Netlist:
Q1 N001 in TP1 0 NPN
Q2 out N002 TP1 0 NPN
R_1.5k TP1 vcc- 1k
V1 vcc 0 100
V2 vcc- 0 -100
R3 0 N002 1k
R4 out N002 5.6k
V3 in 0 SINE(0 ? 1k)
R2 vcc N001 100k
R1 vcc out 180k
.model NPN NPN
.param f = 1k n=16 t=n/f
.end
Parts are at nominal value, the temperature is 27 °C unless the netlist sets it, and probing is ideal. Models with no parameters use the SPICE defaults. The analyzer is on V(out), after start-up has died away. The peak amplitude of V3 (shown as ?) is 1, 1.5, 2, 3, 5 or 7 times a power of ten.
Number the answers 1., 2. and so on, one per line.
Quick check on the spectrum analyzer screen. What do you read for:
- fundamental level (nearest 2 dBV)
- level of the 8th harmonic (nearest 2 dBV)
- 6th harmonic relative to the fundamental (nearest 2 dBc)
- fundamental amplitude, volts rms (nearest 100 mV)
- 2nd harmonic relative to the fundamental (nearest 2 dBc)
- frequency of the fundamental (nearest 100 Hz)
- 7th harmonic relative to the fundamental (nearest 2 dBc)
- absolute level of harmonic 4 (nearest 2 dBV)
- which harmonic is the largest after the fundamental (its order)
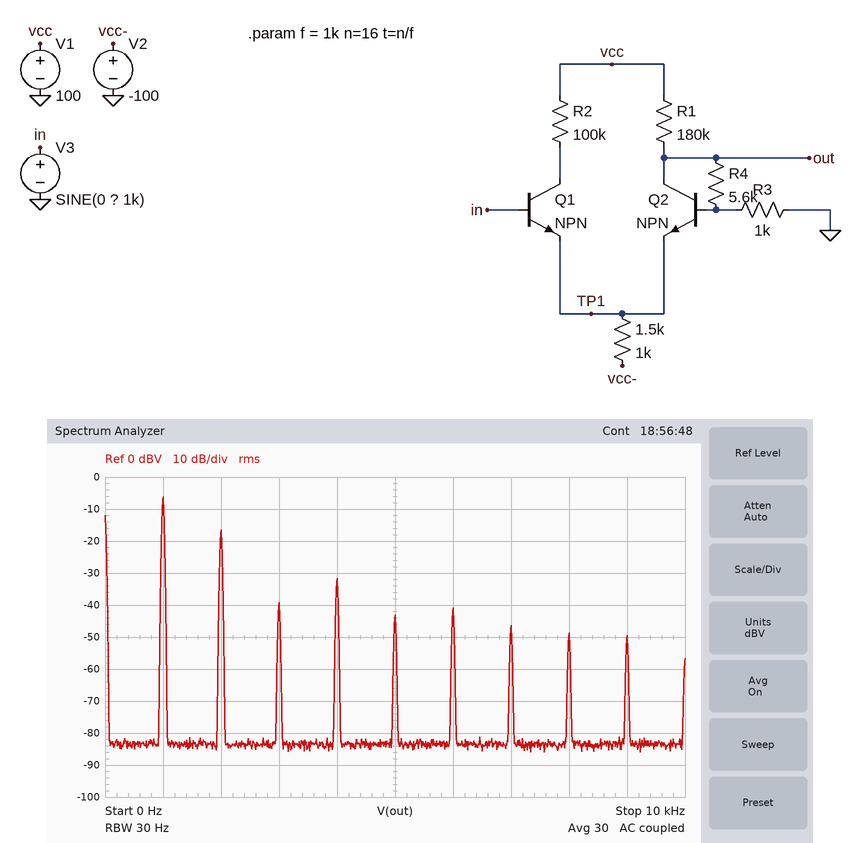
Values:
1. -6 dBV
2. -48 dBV
3. -34 dBc
4. 500 mV
5. -10 dBc
6. 1.0 kHz
7. -40 dBc
8. -32 dBV
9. 2
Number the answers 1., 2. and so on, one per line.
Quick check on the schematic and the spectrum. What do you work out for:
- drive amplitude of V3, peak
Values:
1. 200 mV
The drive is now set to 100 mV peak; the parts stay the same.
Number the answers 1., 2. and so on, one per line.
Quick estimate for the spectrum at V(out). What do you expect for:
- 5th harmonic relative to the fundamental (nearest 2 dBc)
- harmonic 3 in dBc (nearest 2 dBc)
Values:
1. -32 dBc
2. -26 dBc
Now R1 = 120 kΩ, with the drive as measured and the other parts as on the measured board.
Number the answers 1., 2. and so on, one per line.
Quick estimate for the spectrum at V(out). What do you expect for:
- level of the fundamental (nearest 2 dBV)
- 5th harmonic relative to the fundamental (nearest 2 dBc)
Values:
1. -6 dBV
2. -46 dBc
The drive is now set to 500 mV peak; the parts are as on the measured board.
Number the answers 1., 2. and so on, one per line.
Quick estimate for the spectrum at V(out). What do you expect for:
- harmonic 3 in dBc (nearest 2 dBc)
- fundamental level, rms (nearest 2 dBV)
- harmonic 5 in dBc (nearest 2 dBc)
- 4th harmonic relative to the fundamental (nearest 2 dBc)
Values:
1. -52 dBc
2. 2 dBV
3. -46 dBc
4. -24 dBc
